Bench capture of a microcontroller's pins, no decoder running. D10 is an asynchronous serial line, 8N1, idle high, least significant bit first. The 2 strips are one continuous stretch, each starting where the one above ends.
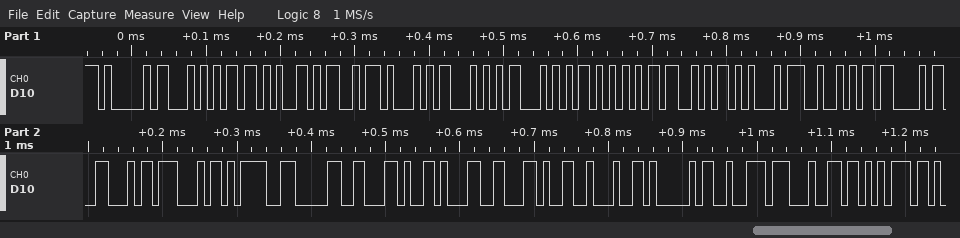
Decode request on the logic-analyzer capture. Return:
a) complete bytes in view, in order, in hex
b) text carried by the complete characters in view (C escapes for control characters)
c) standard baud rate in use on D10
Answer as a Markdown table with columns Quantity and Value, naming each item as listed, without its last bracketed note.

| Quantity | Value |
|---|---|
| complete bytes in view, in order, in hex | 41 54 2B 4D 51 54 54 55 53 45 52 43 46 47 3D 30 2C 31 2C 22 41 72 64 75 |
| text carried by the complete characters in view | "AT+MQTTUSERCFG=0,1,\"Ardu" |
| standard baud rate in use on D10 | 115200 baud |
